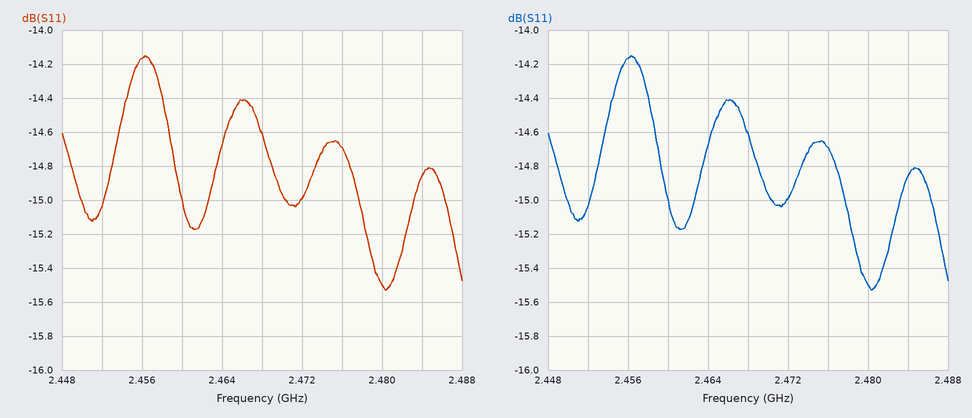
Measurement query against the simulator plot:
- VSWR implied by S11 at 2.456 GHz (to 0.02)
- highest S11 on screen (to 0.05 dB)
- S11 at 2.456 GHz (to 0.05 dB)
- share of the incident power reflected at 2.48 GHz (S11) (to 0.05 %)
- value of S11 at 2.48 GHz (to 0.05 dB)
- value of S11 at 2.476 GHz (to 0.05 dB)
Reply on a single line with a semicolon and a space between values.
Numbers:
1.48; -14.15 dB; -14.15 dB; 2.80 %; -15.50 dB; -14.70 dB
